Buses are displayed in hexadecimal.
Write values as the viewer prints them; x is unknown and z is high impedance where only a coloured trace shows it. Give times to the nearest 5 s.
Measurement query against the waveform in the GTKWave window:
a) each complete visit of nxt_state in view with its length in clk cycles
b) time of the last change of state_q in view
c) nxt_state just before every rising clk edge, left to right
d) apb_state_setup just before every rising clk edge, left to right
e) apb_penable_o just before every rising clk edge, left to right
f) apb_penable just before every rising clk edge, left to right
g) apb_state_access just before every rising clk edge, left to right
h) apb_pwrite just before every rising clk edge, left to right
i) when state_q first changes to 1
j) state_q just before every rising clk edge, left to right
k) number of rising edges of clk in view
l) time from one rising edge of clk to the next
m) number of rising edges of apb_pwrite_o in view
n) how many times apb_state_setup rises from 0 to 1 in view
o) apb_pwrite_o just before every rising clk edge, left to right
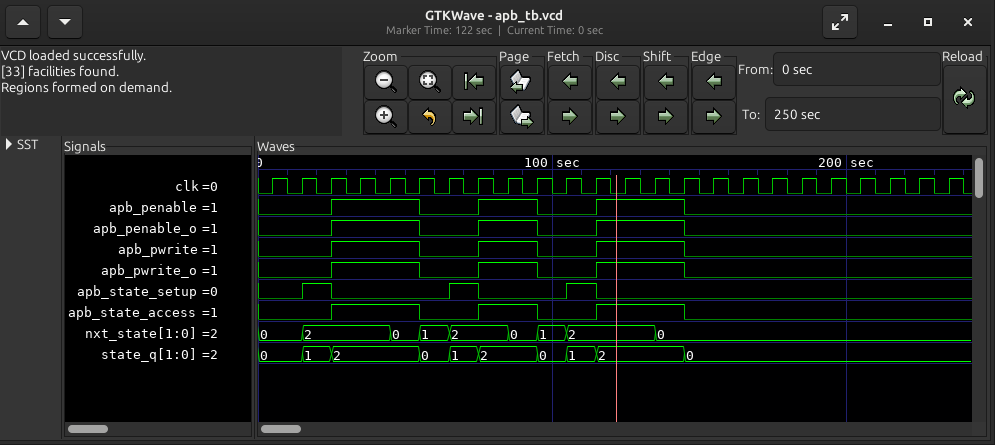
2: 3, 0: 1, 1: 1, 2: 2, 0: 1, 1: 1, 2: 3
145 s
0, 0, 2, 2, 2, 0, 1, 2, 2, 0, 1, 2, 2, 2, 0, 0, 0, 0, 0, 0, 0, 0, 0, 0
0 0 1 0 0 0 0 1 0 0 0 1 0 0 0 0 0 0 0 0 0 0 0 0
0 0 0 1 1 1 0 0 1 1 0 0 1 1 1 0 0 0 0 0 0 0 0 0
0 0 0 1 1 1 0 0 1 1 0 0 1 1 1 0 0 0 0 0 0 0 0 0
0 0 0 1 1 1 0 0 1 1 0 0 1 1 1 0 0 0 0 0 0 0 0 0
0 0 0 1 1 1 0 0 1 1 0 0 1 1 1 0 0 0 0 0 0 0 0 0
15 s
0, 0, 1, 2, 2, 2, 0, 1, 2, 2, 0, 1, 2, 2, 2, 0, 0, 0, 0, 0, 0, 0, 0, 0
24
10 s
3
3
0 0 0 1 1 1 0 0 1 1 0 0 1 1 1 0 0 0 0 0 0 0 0 0
